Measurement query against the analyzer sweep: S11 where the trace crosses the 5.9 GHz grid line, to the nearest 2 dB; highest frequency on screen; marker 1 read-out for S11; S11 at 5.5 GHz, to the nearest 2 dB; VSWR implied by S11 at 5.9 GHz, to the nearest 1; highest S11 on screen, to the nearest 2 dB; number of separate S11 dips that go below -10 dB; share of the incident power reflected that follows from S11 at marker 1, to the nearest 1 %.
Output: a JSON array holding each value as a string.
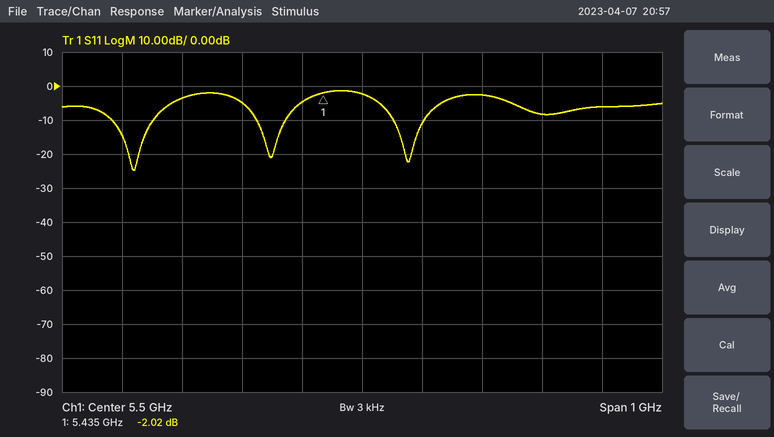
["-6 dB", "6 GHz", "-2.02 dB", "-2 dB", "3", "-2 dB", "3", "63 %"]
